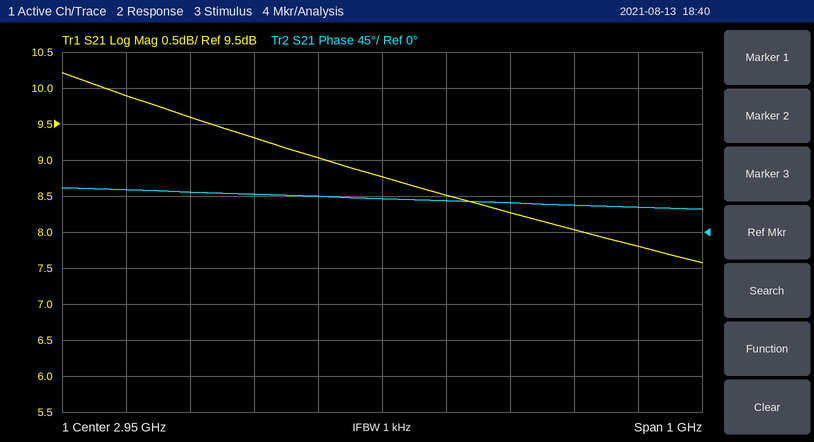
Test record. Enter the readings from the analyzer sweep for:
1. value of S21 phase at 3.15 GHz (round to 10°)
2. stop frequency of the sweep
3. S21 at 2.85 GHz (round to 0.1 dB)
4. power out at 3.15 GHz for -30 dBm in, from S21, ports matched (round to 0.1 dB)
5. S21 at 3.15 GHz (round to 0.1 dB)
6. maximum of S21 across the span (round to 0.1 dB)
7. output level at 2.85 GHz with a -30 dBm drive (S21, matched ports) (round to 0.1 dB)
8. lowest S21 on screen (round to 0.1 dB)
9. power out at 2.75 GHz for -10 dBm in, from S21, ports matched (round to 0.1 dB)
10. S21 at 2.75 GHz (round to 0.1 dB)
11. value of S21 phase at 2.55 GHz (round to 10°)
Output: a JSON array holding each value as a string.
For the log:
["40°", "3.45 GHz", "9.0 dB", "-21.7 dBm", "8.3 dB", "10.2 dB", "-21.0 dBm", "7.6 dB", "-0.7 dBm", "9.3 dB", "50°"]
